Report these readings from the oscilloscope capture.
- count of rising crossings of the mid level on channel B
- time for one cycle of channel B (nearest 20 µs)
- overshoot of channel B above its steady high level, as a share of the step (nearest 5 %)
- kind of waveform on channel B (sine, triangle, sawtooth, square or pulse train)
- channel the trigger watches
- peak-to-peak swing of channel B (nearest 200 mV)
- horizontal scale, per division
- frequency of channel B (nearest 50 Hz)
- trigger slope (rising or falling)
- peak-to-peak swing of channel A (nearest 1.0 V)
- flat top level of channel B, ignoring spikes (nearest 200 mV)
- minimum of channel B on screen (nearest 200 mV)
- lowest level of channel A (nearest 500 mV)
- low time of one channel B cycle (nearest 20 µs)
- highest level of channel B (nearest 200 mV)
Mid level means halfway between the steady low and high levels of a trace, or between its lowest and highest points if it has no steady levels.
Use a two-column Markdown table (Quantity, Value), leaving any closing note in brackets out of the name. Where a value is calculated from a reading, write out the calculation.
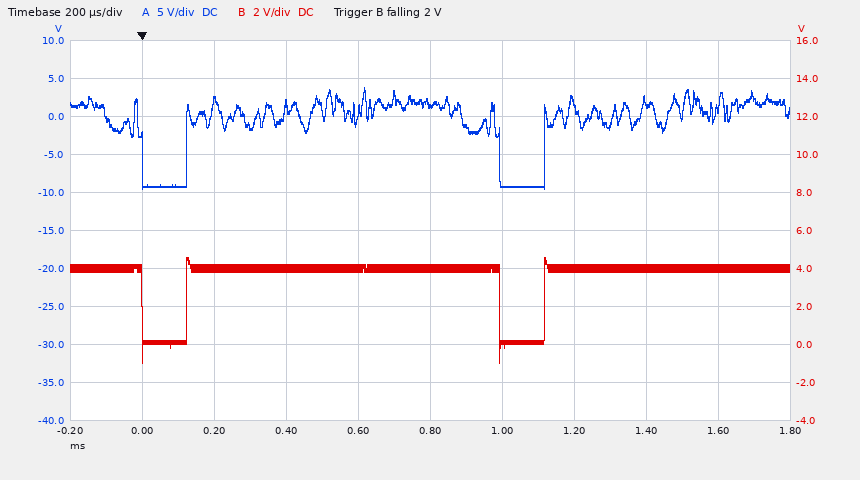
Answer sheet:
| Quantity | Value |
|---|---|
| count of rising crossings of the mid level on channel B | 2 |
| time for one cycle of channel B | 1.00 ms |
| overshoot of channel B above its steady high level, as a share of the step | 15 % |
| kind of waveform on channel B | pulse train |
| channel the trigger watches | channel B |
| peak-to-peak swing of channel B | 4.6 V − (-1.0 V) = 5.6 V |
| horizontal scale, per division | 200 µs |
| frequency of channel B | 1 / 1.00 ms ≈ 1.00 kHz |
| trigger slope | falling |
| peak-to-peak swing of channel A | 13.0 V |
| flat top level of channel B, ignoring spikes | 4.0 V |
| minimum of channel B on screen | -1.0 V |
| lowest level of channel A | -9.5 V |
| low time of one channel B cycle | 120 µs |
| highest level of channel B | 4.6 V |
